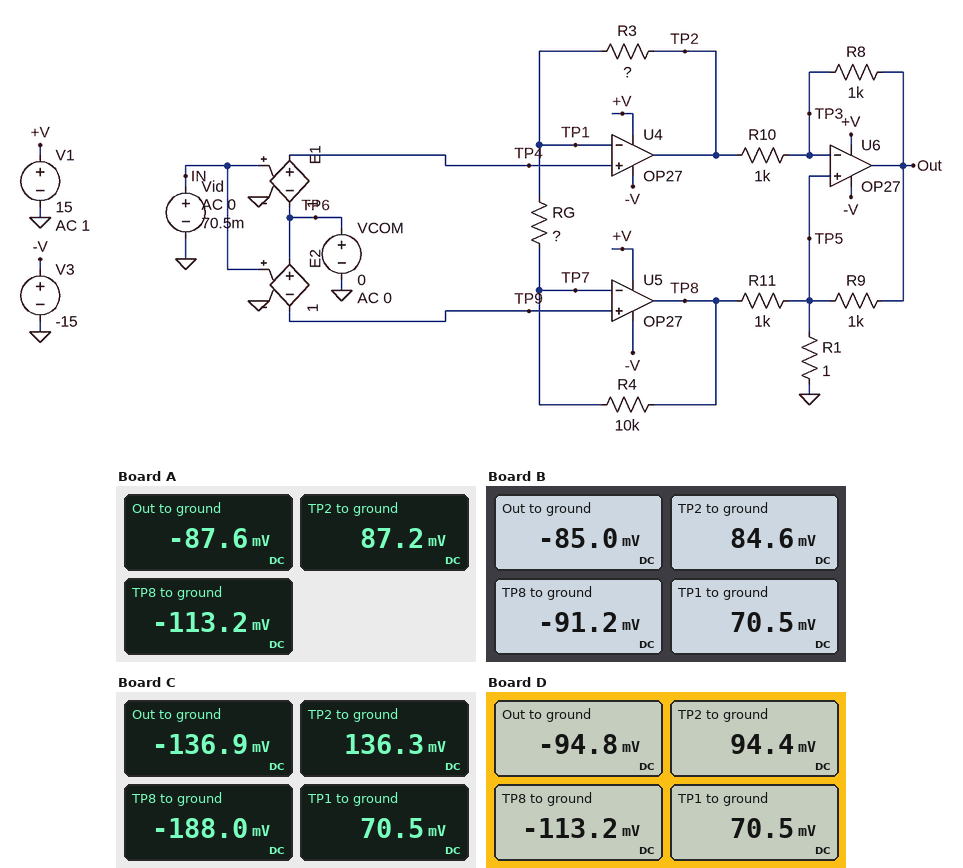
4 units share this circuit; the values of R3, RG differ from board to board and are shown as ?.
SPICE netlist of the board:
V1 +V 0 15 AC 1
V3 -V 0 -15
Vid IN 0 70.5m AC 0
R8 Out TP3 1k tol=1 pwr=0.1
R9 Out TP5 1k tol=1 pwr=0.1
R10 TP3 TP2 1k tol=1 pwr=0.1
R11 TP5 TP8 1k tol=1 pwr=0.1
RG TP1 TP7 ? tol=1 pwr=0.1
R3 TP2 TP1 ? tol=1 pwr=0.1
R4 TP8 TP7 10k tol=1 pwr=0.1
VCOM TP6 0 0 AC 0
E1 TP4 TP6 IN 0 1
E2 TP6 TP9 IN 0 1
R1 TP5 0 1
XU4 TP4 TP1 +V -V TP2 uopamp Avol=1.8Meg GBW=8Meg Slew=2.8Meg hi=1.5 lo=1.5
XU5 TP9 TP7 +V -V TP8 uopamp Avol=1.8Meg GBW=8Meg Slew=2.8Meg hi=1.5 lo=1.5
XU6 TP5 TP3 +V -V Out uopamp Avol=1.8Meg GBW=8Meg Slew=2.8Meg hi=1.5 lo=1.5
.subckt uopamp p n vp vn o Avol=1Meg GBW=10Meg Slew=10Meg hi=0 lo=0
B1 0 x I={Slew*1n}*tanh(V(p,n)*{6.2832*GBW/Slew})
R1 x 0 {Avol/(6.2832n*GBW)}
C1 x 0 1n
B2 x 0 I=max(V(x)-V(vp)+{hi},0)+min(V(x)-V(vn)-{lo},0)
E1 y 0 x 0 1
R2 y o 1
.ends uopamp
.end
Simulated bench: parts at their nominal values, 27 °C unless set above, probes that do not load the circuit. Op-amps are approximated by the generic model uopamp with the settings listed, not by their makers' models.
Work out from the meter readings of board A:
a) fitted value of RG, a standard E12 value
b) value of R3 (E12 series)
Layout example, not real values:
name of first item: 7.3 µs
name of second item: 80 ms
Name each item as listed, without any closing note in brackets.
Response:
fitted value of RG, a standard E12 value: 33 kΩ
value of R3: 3.9 kΩ
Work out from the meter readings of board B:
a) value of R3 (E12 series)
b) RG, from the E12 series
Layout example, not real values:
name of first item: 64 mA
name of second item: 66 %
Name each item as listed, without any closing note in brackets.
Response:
value of R3: 6.8 kΩ
RG, from the E12 series: 68 kΩ
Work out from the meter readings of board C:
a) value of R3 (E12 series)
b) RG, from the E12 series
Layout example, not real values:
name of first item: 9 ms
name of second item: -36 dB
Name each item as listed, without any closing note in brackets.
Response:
value of R3: 5.6 kΩ
RG, from the E12 series: 12 kΩ
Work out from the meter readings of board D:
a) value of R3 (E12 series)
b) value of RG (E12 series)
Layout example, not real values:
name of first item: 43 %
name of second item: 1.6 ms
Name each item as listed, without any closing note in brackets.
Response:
value of R3: 5.6 kΩ
value of RG: 33 kΩ
